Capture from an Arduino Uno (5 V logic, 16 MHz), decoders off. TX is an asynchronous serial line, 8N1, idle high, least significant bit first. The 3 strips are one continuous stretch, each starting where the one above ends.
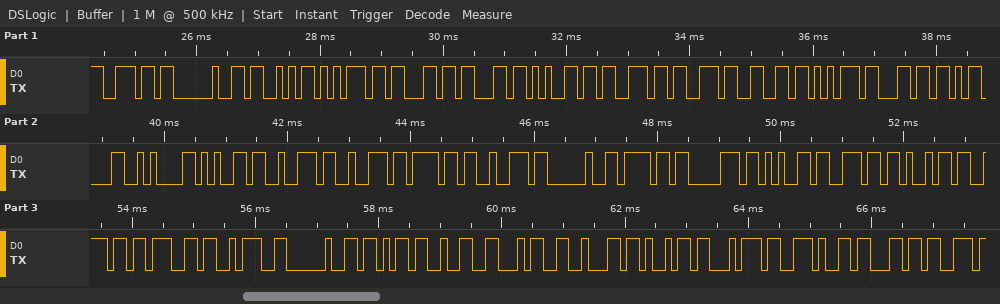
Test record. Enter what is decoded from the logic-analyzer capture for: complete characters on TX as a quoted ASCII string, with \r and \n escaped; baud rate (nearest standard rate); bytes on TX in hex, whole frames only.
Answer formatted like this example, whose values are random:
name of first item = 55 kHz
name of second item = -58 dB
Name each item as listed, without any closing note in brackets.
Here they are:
complete characters on TX as a quoted ASCII string, with \r and \n escaped = "n Successful\r\nerror opening: k24bit.cs"
baud rate = 9600 baud
bytes on TX in hex, whole frames only = 6E 20 53 75 63 63 65 73 73 66 75 6C 0D 0A 65 72 72 6F 72 20 6F 70 65 6E 69 6E 67 3A 20 6B 32 34 62 69 74 2E 63 73
